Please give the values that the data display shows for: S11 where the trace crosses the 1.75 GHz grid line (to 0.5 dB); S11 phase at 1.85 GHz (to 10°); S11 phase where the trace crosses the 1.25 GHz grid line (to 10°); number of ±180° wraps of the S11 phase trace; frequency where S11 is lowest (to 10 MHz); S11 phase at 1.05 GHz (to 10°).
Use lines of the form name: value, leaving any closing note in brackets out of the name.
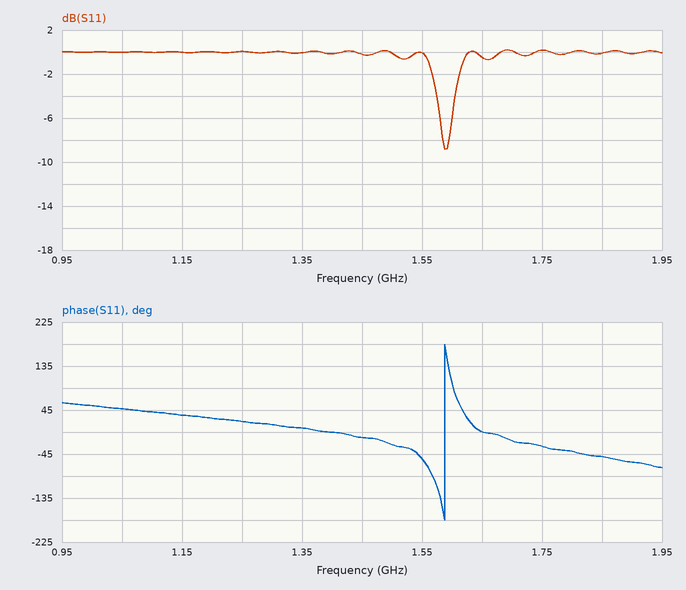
S11 where the trace crosses the 1.75 GHz grid line: 0.0 dB
S11 phase at 1.85 GHz: -50°
S11 phase where the trace crosses the 1.25 GHz grid line: 20°
number of ±180° wraps of the S11 phase trace: 1
frequency where S11 is lowest: 1.59 GHz
S11 phase at 1.05 GHz: 50°
